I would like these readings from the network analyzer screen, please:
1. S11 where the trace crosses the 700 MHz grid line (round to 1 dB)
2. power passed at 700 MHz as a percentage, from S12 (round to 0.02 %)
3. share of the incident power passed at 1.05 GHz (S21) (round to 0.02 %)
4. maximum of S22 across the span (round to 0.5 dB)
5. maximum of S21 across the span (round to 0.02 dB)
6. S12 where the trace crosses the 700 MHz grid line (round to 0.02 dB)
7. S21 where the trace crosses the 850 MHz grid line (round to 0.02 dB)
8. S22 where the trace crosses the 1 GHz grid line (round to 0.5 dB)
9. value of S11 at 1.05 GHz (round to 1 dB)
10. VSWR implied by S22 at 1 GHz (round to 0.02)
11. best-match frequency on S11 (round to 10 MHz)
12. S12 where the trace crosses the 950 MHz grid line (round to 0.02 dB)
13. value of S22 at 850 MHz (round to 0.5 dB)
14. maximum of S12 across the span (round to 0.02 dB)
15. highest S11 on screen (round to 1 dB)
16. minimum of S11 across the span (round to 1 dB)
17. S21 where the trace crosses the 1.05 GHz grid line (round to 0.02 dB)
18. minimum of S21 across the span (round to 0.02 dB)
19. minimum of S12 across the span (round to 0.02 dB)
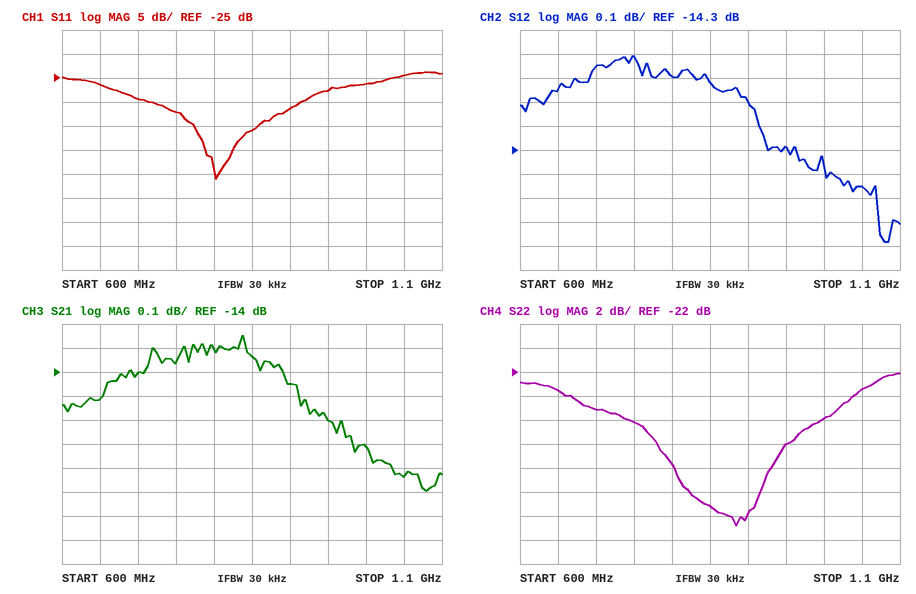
-29 dB
4.02 %
3.60 %
-22.0 dB
-13.84 dB
-13.96 dB
-13.94 dB
-26.0 dB
-24 dB
1.10
800 MHz
-14.28 dB
-33.0 dB
-13.90 dB
-24 dB
-46 dB
-14.44 dB
-14.50 dB
-14.68 dB
